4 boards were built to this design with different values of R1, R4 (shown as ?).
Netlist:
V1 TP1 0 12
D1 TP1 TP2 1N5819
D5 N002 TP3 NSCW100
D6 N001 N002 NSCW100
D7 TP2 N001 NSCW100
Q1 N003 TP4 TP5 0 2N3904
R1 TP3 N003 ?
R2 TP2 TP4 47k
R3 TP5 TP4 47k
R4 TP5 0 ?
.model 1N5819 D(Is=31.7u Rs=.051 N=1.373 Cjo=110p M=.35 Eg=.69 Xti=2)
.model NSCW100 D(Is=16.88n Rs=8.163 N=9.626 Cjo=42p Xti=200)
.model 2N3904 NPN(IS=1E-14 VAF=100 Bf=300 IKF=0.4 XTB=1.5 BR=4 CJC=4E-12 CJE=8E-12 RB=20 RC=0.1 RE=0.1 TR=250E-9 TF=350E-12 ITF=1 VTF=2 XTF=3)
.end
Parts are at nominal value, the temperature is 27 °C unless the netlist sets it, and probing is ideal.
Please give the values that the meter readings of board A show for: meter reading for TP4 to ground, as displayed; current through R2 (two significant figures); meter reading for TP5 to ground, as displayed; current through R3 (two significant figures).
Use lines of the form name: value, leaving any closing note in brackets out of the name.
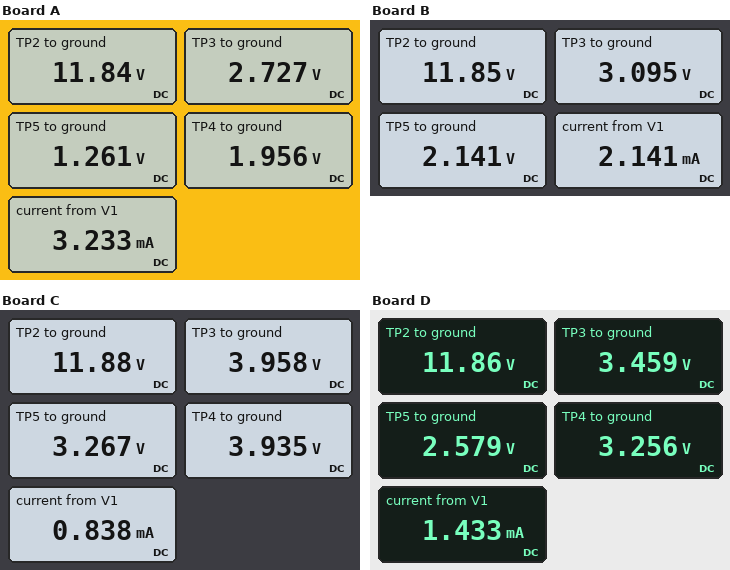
meter reading for TP4 to ground, as displayed: 1.956 V
current through R2: 210 µA
meter reading for TP5 to ground, as displayed: 1.261 V
current through R3: 15 µA
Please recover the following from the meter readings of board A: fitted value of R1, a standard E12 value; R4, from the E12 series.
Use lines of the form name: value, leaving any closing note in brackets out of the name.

fitted value of R1, a standard E12 value: 470 Ω
R4, from the E12 series: 390 Ω
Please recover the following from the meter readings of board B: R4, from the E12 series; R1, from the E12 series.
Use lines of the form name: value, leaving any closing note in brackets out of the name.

R4, from the E12 series: 1 kΩ
R1, from the E12 series: 470 Ω
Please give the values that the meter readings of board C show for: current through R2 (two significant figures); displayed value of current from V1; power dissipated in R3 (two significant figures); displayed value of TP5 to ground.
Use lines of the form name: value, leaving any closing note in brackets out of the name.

current through R2: 170 µA
displayed value of current from V1: 0.838 mA
power dissipated in R3: 9.5 µW
displayed value of TP5 to ground: 3.267 V
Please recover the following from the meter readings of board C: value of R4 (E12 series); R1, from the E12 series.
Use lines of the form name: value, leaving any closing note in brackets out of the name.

value of R4: 3.9 kΩ
R1, from the E12 series: 1 kΩ
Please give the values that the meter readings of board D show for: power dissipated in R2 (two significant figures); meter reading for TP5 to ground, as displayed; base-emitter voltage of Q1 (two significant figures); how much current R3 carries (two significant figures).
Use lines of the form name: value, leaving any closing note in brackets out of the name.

power dissipated in R2: 1.6 mW
meter reading for TP5 to ground, as displayed: 2.579 V
base-emitter voltage of Q1: 680 mV
how much current R3 carries: 14 µA
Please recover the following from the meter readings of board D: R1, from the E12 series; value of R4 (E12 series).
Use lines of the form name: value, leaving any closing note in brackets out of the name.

R1, from the E12 series: 680 Ω
value of R4: 1.8 kΩ
